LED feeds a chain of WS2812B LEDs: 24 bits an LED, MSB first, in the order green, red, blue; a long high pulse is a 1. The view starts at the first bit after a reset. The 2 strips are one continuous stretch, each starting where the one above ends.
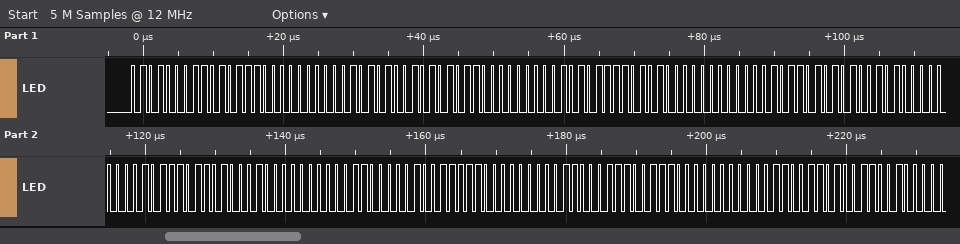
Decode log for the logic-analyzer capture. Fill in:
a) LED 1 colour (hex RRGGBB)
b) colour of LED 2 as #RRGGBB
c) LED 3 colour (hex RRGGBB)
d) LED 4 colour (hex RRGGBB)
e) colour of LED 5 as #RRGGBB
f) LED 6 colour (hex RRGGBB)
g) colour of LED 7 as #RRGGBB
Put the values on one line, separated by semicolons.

#AE5100; #AB5400; #A85700; #A55A00; #A25D00; #9F6000; #9C6300
